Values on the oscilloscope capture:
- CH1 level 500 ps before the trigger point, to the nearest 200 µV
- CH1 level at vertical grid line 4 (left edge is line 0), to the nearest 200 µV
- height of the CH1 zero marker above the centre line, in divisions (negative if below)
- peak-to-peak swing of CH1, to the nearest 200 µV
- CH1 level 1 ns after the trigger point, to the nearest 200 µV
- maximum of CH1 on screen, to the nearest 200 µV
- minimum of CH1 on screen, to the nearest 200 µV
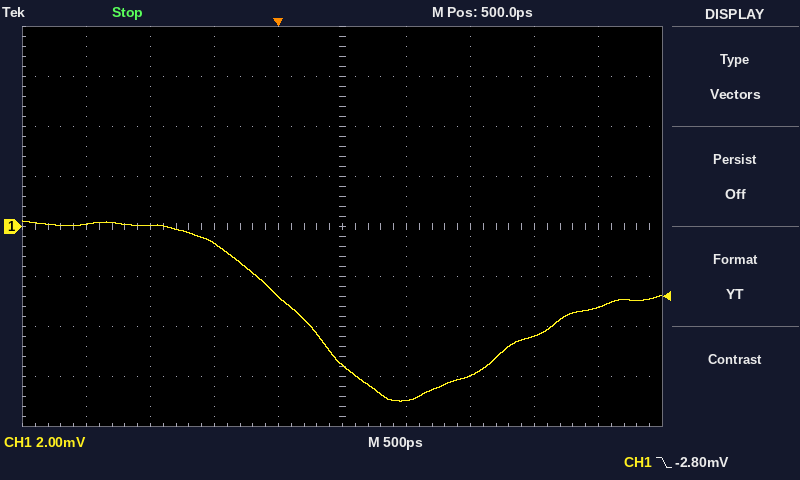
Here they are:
-600 µV
-2.8 mV
0.0 div
7.2 mV
-7.0 mV
200 µV
-7.0 mV
